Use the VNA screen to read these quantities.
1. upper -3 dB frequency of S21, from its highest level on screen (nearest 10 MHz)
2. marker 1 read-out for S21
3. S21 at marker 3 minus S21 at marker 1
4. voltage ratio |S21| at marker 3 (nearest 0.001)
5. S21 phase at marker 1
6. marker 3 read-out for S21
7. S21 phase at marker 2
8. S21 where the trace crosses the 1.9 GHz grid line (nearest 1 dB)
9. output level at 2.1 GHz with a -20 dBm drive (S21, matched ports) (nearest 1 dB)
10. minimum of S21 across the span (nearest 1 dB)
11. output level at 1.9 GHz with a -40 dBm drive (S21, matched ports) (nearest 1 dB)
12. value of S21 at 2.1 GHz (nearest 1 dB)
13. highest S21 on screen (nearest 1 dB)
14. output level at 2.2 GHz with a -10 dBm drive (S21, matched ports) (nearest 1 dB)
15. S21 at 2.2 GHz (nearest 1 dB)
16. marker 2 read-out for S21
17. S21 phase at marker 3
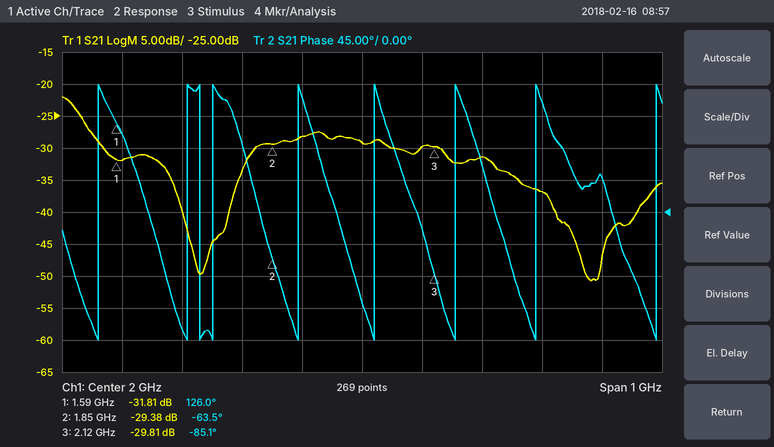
1.53 GHz
-31.81 dB
2.00 dB
0.032
126.0°
-29.81 dB
-63.5°
-28 dB
-50 dBm
-51 dB
-68 dBm
-30 dB
-22 dB
-41 dBm
-31 dB
-29.38 dB
-85.1°
